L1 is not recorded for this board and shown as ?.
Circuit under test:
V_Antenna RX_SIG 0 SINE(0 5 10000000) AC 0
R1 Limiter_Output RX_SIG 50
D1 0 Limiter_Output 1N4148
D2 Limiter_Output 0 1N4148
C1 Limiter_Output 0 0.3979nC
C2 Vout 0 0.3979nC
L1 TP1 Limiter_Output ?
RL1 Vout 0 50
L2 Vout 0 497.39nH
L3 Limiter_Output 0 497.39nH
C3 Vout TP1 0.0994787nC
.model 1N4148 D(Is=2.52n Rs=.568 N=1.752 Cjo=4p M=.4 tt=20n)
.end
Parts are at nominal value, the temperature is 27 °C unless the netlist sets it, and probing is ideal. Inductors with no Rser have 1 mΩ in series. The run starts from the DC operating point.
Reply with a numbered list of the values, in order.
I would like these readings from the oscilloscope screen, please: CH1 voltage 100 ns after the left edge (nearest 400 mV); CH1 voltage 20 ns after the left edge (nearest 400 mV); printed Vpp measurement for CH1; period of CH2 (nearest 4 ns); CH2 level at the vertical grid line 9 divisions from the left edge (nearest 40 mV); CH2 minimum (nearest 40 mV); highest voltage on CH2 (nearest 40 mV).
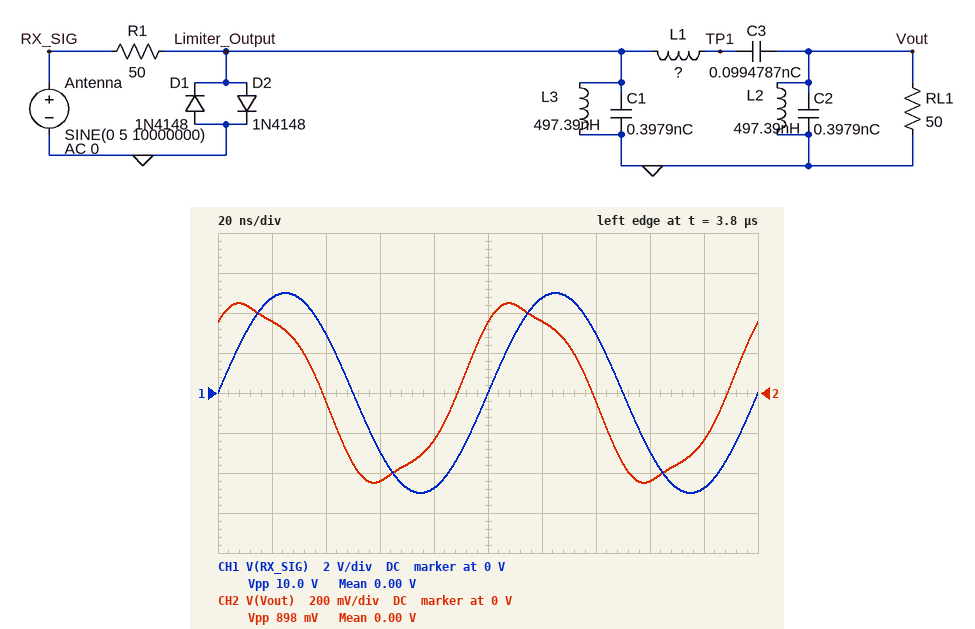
1. 0 V
2. 4.8 V
3. 10.0 V
4. 100 ns
5. -240 mV
6. -440 mV
7. 440 mV
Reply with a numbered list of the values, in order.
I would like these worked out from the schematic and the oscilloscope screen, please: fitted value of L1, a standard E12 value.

1. 820 nH
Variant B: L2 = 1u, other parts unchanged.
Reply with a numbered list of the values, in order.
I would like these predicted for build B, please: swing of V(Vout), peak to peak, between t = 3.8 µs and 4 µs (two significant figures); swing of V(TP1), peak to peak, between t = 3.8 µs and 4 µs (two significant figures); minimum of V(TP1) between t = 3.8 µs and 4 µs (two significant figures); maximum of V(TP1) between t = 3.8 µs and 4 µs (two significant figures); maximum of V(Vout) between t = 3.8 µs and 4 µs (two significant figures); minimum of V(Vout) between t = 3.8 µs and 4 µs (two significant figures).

1. 660 mV
2. 3.0 V
3. -1.5 V
4. 1.5 V
5. 330 mV
6. -330 mV
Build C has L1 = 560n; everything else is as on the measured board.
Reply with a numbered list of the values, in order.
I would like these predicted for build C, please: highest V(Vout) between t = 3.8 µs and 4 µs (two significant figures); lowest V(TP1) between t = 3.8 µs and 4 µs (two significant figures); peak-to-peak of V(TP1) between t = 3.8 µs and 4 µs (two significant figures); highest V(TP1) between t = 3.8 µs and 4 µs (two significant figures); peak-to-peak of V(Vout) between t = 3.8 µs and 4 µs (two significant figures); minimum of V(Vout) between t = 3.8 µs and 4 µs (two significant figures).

1. 440 mV
2. -1.7 V
3. 3.4 V
4. 1.7 V
5. 880 mV
6. -440 mV
